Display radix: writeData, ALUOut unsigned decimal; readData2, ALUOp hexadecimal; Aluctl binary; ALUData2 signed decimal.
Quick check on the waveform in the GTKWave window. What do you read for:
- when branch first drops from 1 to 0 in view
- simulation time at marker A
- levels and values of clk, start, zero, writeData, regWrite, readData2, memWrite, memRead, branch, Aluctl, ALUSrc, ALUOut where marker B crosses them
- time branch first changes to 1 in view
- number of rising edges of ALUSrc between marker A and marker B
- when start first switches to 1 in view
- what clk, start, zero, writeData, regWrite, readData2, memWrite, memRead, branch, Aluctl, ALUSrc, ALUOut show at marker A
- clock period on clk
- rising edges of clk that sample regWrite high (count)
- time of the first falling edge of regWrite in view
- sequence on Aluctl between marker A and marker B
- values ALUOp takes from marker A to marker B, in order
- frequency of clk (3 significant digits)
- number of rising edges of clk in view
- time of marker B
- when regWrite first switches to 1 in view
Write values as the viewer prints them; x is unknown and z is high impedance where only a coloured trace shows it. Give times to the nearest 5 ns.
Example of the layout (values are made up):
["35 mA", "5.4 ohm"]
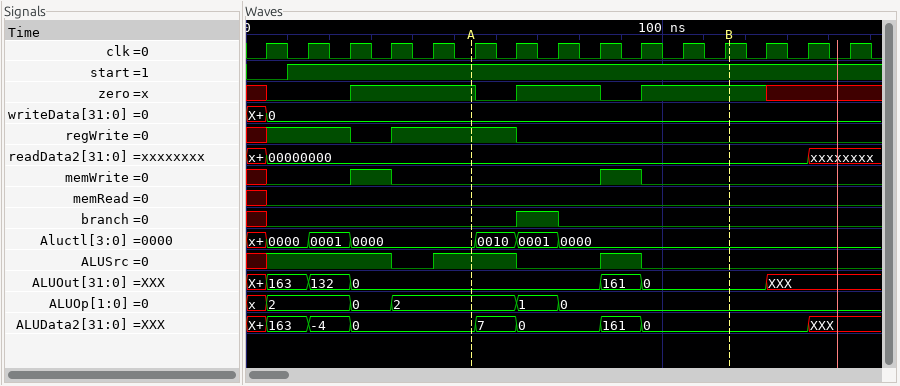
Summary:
["75 ns", "55 ns", "clk=1, start=1, zero=1, writeData=0, regWrite=0, readData2=00000000, memWrite=0, memRead=0, branch=0, Aluctl=0000, ALUSrc=0, ALUOut=0", "65 ns", "1", "10 ns", "clk=0, start=1, zero=1, writeData=0, regWrite=1, readData2=00000000, memWrite=0, memRead=0, branch=0, Aluctl=0000, ALUSrc=1, ALUOut=0", "10 ns", "5", "25 ns", "0000, 0010, 0001, 0000", "2, 1, 0", "100 MHz", "15", "115 ns", "5 ns"]
